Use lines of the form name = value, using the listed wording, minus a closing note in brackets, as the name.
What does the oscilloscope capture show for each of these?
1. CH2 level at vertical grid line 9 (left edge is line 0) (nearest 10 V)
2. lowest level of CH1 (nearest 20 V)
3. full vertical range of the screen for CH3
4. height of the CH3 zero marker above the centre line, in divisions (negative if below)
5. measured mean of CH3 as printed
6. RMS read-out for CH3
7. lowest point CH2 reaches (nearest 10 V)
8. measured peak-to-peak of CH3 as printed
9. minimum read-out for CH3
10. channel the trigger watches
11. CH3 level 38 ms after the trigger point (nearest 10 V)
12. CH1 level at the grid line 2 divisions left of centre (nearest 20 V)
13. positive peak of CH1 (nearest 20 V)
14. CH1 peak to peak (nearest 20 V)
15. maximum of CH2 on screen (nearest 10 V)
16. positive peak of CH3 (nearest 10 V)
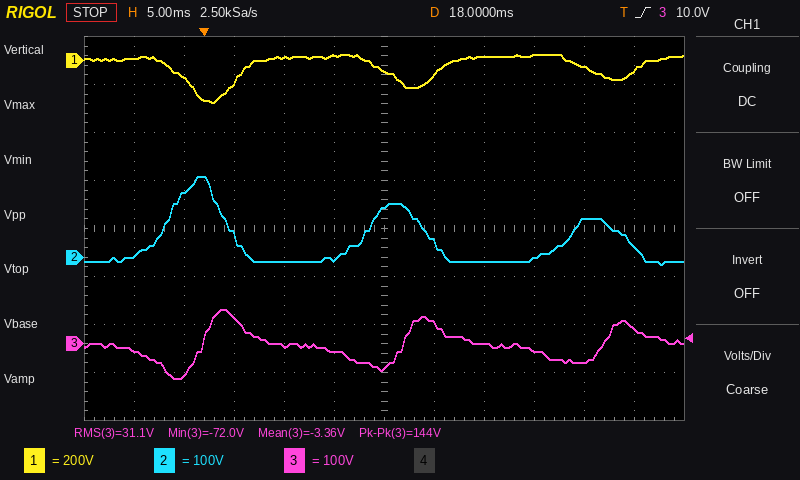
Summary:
CH2 level at vertical grid line 9 (left edge is line 0) = 0 V
lowest level of CH1 = -180 V
full vertical range of the screen for CH3 = 800 V
height of the CH3 zero marker above the centre line, in divisions = -2.4 div
measured mean of CH3 as printed = -3.36 V
RMS read-out for CH3 = 31.1 V
lowest point CH2 reaches = -20 V
measured peak-to-peak of CH3 as printed = 144 V
minimum read-out for CH3 = -72.0 V
channel the trigger watches = CH3
CH3 level 38 ms after the trigger point = -40 V
CH1 level at the grid line 2 divisions left of centre = 20 V
positive peak of CH1 = 20 V
CH1 peak to peak = 200 V
maximum of CH2 on screen = 170 V
positive peak of CH3 = 70 V
